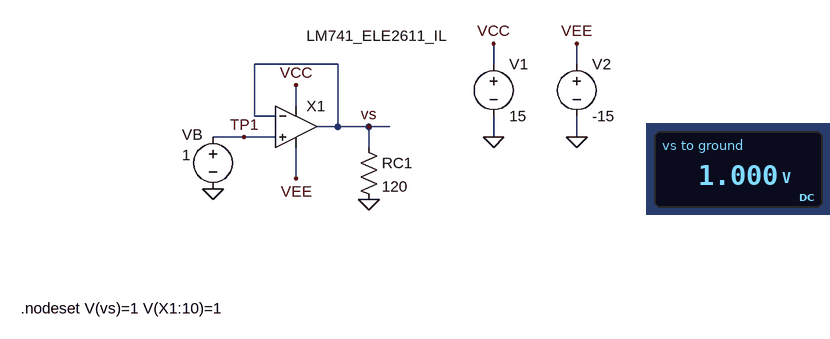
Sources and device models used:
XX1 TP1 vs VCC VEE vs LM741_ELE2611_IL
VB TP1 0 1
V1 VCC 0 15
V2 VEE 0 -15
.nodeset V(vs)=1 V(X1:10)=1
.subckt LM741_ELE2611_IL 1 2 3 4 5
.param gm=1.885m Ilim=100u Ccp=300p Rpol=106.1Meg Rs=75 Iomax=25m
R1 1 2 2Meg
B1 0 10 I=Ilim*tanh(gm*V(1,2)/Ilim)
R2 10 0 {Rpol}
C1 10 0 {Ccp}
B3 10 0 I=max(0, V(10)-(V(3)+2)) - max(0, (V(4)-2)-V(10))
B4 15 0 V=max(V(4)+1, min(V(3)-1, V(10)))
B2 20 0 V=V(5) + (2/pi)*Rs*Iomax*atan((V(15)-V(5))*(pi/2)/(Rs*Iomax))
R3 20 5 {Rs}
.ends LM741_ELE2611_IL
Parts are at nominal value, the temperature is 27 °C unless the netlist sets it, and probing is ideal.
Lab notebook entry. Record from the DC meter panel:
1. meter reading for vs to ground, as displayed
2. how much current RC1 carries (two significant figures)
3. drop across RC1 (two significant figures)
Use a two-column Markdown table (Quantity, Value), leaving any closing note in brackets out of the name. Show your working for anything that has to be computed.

| Quantity | Value |
|---|---|
| meter reading for vs to ground, as displayed | 1.000 V |
| how much current RC1 carries | (1 V) / 120 Ω = 8.3 mA |
| drop across RC1 | 1 V = 1.0 V |
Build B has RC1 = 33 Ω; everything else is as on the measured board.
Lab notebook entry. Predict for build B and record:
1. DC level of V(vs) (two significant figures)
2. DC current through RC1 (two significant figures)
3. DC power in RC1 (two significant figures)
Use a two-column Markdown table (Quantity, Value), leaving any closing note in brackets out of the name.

| Quantity | Value |
|---|---|
| DC level of V(vs) | 780 mV |
| DC current through RC1 | 24 mA |
| DC power in RC1 | 18 mW |
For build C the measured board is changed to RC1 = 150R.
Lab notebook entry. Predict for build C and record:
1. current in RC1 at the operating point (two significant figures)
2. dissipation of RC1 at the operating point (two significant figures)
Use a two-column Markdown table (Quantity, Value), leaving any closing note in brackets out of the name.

| Quantity | Value |
|---|---|
| current in RC1 at the operating point | 6.7 mA |
| dissipation of RC1 at the operating point | 6.7 mW |
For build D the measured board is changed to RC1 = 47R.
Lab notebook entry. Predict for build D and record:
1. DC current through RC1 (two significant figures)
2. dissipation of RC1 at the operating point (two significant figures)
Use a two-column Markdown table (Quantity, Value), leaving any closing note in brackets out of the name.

| Quantity | Value |
|---|---|
| DC current through RC1 | 21 mA |
| dissipation of RC1 at the operating point | 21 mW |
